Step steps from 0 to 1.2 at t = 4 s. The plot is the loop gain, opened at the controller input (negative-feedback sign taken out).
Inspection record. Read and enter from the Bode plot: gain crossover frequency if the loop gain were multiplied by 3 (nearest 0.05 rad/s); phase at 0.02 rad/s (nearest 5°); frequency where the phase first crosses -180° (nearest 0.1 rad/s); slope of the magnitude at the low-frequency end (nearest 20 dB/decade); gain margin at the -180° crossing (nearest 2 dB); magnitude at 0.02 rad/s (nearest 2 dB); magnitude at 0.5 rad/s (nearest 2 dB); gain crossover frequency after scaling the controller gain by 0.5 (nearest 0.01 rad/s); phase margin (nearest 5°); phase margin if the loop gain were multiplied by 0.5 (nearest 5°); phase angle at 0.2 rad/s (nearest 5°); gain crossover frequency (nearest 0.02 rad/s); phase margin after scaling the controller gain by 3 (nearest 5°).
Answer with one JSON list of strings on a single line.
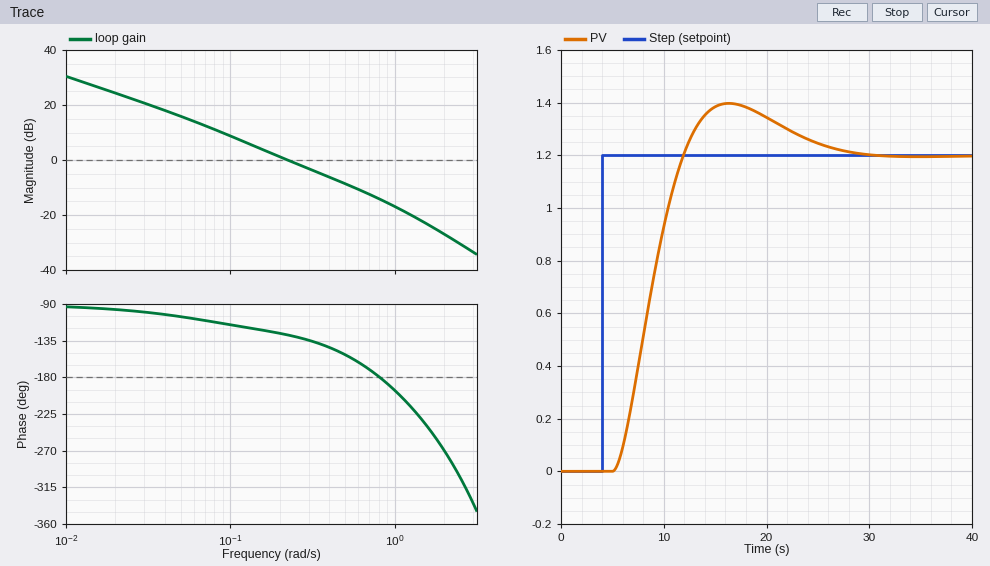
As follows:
["0.55 rad/s", "-95°", "0.8 rad/s", "-20 dB/decade", "14 dB", "24 dB", "-8 dB", "0.13 rad/s", "50°", "60°", "-125°", "0.22 rad/s", "25°"]
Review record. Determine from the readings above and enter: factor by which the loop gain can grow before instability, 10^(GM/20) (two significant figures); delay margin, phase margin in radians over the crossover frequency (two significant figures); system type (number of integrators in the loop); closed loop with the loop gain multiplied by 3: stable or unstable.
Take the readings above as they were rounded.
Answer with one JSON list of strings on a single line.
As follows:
["5.0", "4.0 s", "1", "stable"]
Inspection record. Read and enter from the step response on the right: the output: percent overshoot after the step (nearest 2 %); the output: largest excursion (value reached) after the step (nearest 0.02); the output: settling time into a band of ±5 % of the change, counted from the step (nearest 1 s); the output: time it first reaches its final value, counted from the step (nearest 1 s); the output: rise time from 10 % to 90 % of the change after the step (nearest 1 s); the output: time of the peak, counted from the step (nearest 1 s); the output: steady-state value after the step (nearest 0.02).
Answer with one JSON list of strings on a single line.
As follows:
["16 %", "1.40", "20 s", "8 s", "5 s", "12 s", "1.20"]
